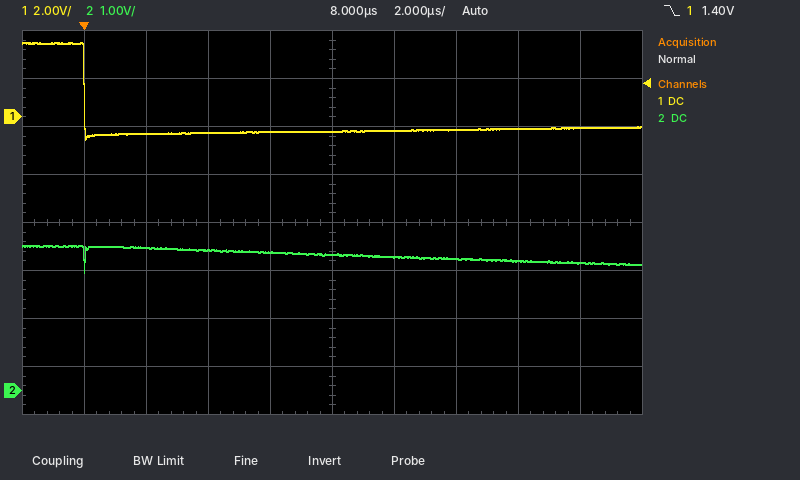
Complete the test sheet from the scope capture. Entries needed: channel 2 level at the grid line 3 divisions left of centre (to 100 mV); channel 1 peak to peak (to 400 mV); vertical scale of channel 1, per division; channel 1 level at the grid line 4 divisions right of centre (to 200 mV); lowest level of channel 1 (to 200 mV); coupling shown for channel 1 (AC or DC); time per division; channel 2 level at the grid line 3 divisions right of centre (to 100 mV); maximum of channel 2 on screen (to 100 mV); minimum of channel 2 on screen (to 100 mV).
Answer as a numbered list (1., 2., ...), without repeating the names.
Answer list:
1. 3.0 V
2. 4.0 V
3. 2 V
4. -400 mV
5. -1.0 V
6. DC
7. 2 µs
8. 2.7 V
9. 3.0 V
10. 2.5 V
